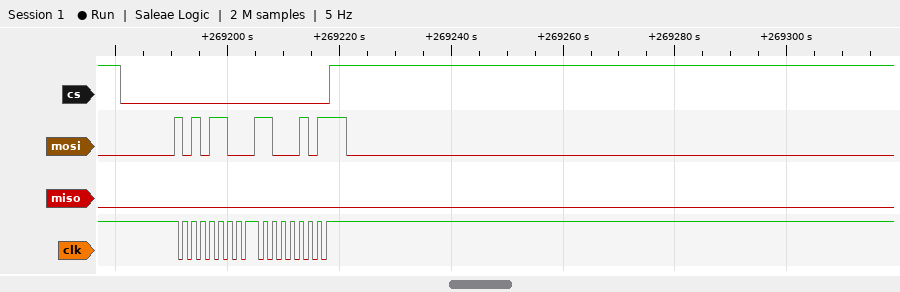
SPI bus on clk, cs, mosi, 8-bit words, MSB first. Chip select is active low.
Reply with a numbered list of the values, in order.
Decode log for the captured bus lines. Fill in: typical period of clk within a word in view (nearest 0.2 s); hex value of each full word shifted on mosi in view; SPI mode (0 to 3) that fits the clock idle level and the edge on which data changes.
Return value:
1. 1.6 s
2. AC, C5
3. 2
